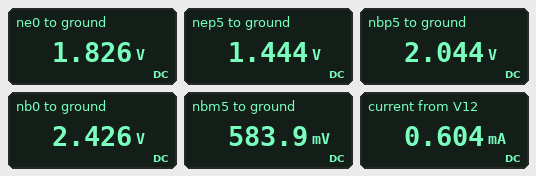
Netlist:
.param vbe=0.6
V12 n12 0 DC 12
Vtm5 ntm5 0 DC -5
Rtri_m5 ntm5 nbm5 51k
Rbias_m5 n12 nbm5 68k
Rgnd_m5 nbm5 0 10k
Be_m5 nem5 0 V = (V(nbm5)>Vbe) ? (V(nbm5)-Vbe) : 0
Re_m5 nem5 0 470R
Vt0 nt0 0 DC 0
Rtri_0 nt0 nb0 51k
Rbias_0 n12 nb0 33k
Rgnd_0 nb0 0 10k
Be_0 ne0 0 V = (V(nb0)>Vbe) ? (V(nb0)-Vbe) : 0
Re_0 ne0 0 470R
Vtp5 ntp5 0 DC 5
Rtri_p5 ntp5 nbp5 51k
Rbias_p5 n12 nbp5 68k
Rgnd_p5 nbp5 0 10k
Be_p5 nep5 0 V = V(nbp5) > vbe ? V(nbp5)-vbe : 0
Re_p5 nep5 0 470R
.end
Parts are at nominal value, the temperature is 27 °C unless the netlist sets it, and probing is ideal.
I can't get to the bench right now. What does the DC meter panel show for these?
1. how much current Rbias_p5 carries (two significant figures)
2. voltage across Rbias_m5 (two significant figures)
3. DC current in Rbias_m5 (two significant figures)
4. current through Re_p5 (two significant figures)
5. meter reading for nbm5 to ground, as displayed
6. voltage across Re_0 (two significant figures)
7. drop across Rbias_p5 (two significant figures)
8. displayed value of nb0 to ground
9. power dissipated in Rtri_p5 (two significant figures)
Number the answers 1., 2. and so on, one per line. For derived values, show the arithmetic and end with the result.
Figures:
1. (12 V - 2.044 V) / 68 kΩ = 150 µA
2. 12 V - 583.9 mV = 11 V
3. (12 V - 583.9 mV) / 68 kΩ = 170 µA
4. (1.444 V) / 470 Ω = 3.1 mA
5. 583.9 mV
6. 1.826 V = 1.8 V
7. 12 V - 2.044 V = 10 V
8. 2.426 V
9. (5 V - 2.044 V)^2 / 51 kΩ = 170 µW
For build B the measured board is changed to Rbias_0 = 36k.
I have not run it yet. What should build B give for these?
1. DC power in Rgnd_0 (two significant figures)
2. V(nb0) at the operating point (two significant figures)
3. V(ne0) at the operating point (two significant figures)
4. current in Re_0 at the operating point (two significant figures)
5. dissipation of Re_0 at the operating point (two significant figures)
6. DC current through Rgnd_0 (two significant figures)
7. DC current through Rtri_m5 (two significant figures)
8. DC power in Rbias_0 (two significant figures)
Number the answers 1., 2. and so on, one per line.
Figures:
1. 510 µW
2. 2.3 V
3. 1.7 V
4. 3.5 mA
5. 5.9 mW
6. 230 µA
7. 110 µA
8. 2.6 mW
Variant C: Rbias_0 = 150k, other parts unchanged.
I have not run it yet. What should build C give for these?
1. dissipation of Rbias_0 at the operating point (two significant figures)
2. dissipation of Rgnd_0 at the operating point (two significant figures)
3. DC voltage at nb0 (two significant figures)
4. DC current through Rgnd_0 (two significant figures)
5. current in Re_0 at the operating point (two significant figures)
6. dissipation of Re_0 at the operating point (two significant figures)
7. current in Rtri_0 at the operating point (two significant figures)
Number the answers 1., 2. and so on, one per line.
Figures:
1. 860 µW
2. 40 µW
3. 630 mV
4. 63 µA
5. 71 µA
6. 2.4 µW
7. 12 µA
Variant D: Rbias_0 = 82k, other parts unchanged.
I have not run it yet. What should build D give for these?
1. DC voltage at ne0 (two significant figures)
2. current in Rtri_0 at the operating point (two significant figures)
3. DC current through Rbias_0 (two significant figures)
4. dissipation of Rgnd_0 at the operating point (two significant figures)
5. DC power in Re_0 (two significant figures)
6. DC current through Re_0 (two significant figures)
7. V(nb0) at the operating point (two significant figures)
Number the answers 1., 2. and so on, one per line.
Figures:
1. 510 mV
2. 22 µA
3. 130 µA
4. 120 µW
5. 550 µW
6. 1.1 mA
7. 1.1 V
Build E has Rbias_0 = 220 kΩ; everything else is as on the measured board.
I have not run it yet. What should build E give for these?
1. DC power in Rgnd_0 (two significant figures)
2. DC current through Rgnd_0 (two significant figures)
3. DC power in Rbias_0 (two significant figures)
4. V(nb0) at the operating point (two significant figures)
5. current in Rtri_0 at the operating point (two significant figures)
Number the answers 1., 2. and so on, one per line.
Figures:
1. 19 µW
2. 44 µA
3. 610 µW
4. 440 mV
5. 8.6 µA
